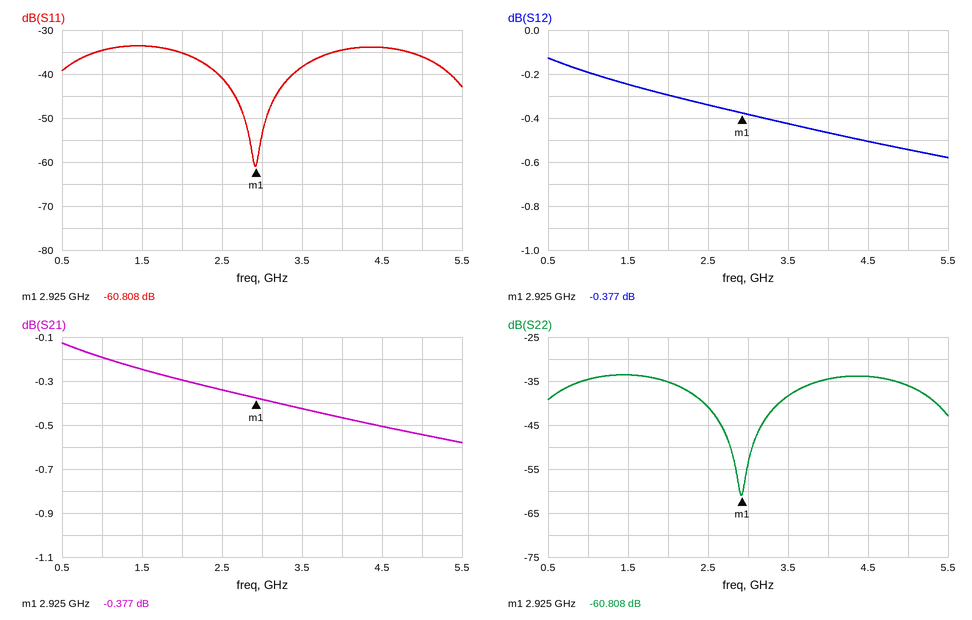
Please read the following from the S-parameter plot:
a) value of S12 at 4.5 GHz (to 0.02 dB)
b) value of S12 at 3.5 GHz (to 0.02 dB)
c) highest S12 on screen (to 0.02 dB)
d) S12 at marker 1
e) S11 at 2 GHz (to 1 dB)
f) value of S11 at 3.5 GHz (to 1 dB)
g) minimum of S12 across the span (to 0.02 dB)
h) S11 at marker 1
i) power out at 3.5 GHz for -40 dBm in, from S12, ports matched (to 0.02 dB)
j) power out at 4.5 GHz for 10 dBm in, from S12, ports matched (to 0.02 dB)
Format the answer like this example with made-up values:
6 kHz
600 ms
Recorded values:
-0.50 dB
-0.42 dB
-0.12 dB
-0.377 dB
-35 dB
-38 dB
-0.58 dB
-60.808 dB
-40.42 dBm
9.50 dBm
